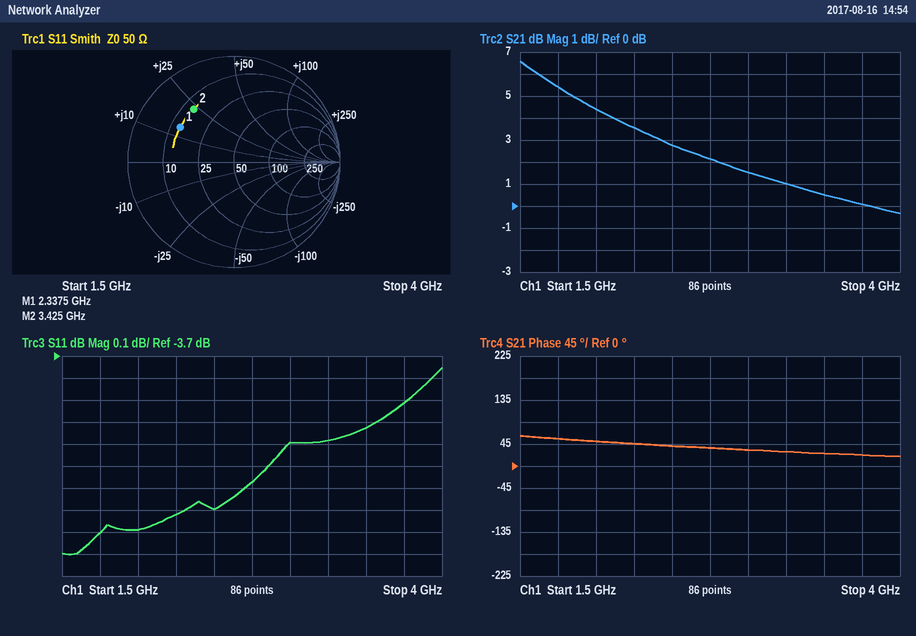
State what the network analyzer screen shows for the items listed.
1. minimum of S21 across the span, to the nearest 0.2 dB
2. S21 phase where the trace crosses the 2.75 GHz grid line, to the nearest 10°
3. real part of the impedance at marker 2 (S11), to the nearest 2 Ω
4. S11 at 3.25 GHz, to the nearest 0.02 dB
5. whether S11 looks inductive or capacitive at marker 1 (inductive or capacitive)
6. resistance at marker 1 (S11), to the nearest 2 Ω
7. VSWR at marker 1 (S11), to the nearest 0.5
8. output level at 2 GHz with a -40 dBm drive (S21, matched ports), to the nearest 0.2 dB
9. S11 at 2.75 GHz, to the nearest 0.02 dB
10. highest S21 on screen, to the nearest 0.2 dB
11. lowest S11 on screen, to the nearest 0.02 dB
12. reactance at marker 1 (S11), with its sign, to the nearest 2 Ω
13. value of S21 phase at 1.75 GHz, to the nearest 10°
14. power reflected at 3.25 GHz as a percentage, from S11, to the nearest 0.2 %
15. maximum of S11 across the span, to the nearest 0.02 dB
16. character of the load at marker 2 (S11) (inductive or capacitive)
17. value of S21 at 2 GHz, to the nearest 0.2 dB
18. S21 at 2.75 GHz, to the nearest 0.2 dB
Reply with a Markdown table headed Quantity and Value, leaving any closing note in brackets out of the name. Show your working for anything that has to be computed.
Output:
| Quantity | Value |
|---|---|
| minimum of S21 across the span, to the nearest 0.2 dB | -0.4 dB |
| S21 phase where the trace crosses the 2.75 GHz grid line, to the nearest 10° | 40° |
| real part of the impedance at marker 2 (S11), to the nearest 2 Ω | 14 Ω |
| S11 at 3.25 GHz, to the nearest 0.02 dB | -4.08 dB |
| whether S11 looks inductive or capacitive at marker 1 | inductive |
| resistance at marker 1 (S11), to the nearest 2 Ω | 14 Ω |
| VSWR at marker 1 (S11), to the nearest 0.5 | 4.0 |
| output level at 2 GHz with a -40 dBm drive (S21, matched ports), to the nearest 0.2 dB | -40 dBm + (4.4 dB) = -35.6 dBm |
| S11 at 2.75 GHz, to the nearest 0.02 dB | -4.28 dB |
| highest S21 on screen, to the nearest 0.2 dB | 6.6 dB |
| lowest S11 on screen, to the nearest 0.02 dB | -4.60 dB |
| reactance at marker 1 (S11), with its sign, to the nearest 2 Ω | +14 Ω |
| value of S21 phase at 1.75 GHz, to the nearest 10° | 60° |
| power reflected at 3.25 GHz as a percentage, from S11, to the nearest 0.2 % | 10^(-4.08/10) ≈ 39.1 %, so 39.0 % to the nearest 0.2 % |
| maximum of S11 across the span, to the nearest 0.02 dB | -3.76 dB |
| character of the load at marker 2 (S11) | inductive |
| value of S21 at 2 GHz, to the nearest 0.2 dB | 4.4 dB |
| S21 at 2.75 GHz, to the nearest 0.2 dB | 2.2 dB |
